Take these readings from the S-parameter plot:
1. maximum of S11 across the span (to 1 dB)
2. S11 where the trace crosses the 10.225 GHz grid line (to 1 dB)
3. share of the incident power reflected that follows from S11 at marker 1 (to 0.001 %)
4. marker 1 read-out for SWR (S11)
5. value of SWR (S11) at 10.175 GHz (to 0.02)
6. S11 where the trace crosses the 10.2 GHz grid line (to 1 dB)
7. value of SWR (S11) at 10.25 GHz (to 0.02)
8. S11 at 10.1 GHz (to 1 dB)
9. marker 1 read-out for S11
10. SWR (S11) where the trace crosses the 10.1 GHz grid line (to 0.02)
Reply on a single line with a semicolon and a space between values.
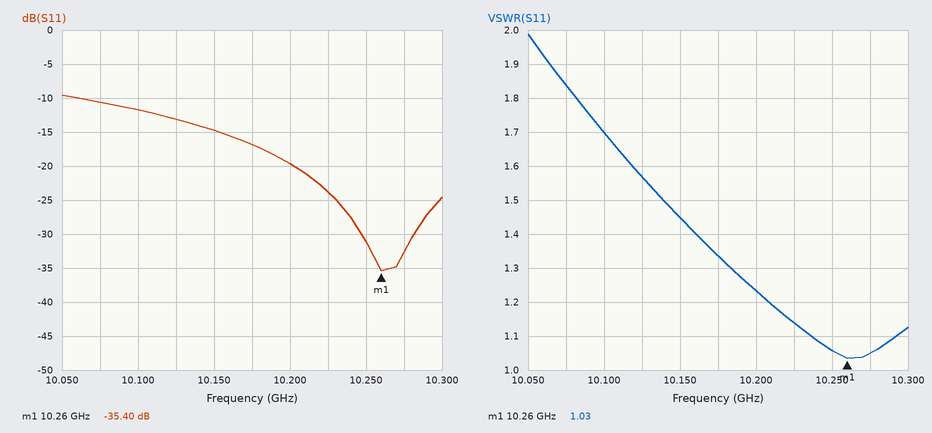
-10 dB; -24 dB; 0.029 %; 1.03; 1.34; -20 dB; 1.06; -12 dB; -35.40 dB; 1.70
